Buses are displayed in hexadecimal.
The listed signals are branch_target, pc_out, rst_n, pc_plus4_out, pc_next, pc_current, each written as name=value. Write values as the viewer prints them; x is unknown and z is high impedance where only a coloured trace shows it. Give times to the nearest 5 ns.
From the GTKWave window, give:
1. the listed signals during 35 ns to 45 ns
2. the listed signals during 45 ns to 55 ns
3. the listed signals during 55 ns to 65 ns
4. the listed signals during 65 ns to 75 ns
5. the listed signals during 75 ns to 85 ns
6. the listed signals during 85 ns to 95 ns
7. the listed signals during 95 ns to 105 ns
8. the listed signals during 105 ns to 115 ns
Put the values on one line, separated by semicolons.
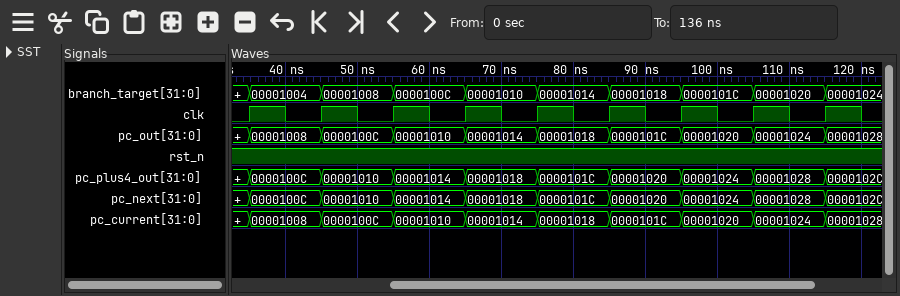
branch_target=00001004, pc_out=00001008, rst_n=1, pc_plus4_out=0000100C, pc_next=0000100C, pc_current=00001008; branch_target=00001008, pc_out=0000100C, rst_n=1, pc_plus4_out=00001010, pc_next=00001010, pc_current=0000100C; branch_target=0000100C, pc_out=00001010, rst_n=1, pc_plus4_out=00001014, pc_next=00001014, pc_current=00001010; branch_target=00001010, pc_out=00001014, rst_n=1, pc_plus4_out=00001018, pc_next=00001018, pc_current=00001014; branch_target=00001014, pc_out=00001018, rst_n=1, pc_plus4_out=0000101C, pc_next=0000101C, pc_current=00001018; branch_target=00001018, pc_out=0000101C, rst_n=1, pc_plus4_out=00001020, pc_next=00001020, pc_current=0000101C; branch_target=0000101C, pc_out=00001020, rst_n=1, pc_plus4_out=00001024, pc_next=00001024, pc_current=00001020; branch_target=00001020, pc_out=00001024, rst_n=1, pc_plus4_out=00001028, pc_next=00001028, pc_current=00001024
